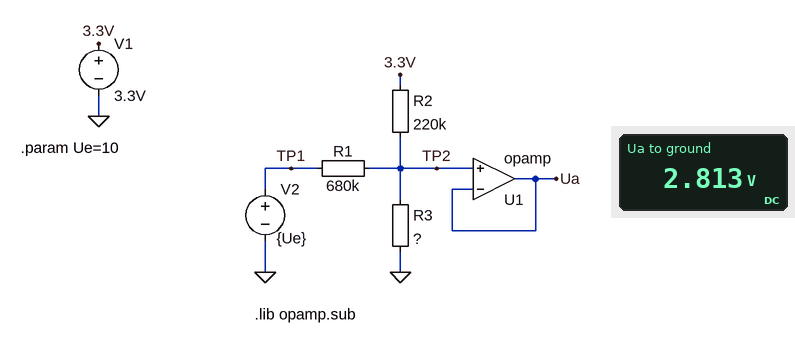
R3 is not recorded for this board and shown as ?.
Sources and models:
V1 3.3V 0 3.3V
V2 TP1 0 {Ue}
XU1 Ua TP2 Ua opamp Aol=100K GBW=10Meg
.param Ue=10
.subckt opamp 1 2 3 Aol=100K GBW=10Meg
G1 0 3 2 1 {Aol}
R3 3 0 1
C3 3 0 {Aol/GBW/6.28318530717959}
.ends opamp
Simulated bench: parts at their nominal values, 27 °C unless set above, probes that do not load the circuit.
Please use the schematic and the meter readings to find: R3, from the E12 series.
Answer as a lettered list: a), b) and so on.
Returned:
a) 220 kΩ
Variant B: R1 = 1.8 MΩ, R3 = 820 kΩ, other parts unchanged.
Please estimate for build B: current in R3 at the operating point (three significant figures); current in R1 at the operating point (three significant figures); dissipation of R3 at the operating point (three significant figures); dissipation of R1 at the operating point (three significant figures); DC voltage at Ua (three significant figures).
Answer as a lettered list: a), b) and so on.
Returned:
a) 3.97 µA
b) 3.75 µA
c) 12.9 µW
d) 25.3 µW
e) 3.25 V
